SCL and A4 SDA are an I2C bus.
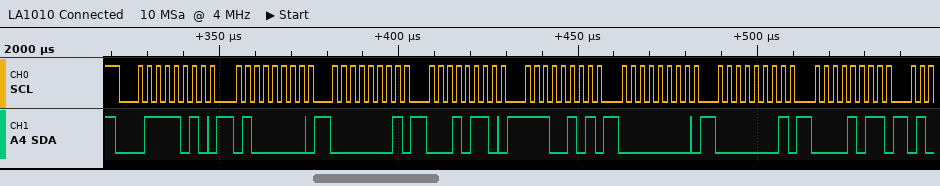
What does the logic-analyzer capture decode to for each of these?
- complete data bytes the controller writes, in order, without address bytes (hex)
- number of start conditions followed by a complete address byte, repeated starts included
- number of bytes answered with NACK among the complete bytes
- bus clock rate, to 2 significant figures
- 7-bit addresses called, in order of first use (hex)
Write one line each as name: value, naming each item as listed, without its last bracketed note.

complete data bytes the controller writes, in order, without address bytes: 40 01 16 E5 00 01 0B
number of start conditions followed by a complete address byte, repeated starts included: 1
number of bytes answered with NACK among the complete bytes: 0
bus clock rate, to 2 significant figures: 400 kHz
7-bit addresses called, in order of first use: 0x3D
